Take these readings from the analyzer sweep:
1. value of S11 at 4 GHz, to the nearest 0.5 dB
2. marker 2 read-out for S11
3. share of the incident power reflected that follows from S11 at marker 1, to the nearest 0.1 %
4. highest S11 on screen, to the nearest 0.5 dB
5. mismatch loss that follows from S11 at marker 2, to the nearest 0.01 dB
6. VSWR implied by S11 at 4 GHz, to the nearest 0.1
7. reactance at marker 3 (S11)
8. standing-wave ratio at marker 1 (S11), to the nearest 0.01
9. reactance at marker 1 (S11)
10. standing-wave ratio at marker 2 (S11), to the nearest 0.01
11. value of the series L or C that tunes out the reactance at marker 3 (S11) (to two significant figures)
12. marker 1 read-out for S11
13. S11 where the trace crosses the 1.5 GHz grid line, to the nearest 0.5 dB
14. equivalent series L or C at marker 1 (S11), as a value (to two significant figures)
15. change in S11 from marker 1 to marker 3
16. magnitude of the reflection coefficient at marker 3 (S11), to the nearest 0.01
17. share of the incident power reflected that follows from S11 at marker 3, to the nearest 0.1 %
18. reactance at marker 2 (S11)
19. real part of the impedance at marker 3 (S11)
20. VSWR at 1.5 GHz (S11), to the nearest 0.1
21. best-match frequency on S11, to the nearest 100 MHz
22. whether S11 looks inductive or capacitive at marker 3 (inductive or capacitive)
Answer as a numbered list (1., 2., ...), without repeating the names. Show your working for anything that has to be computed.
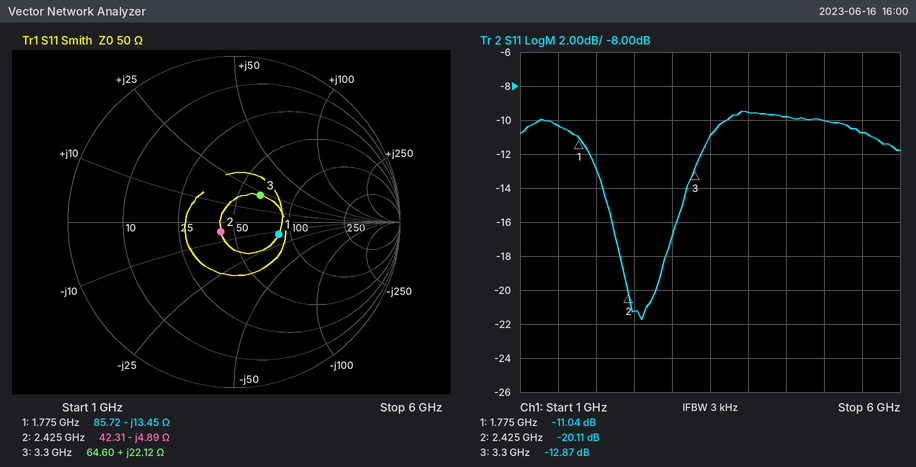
1. -9.5 dB
2. -20.11 dB
3. 10^(-11.04/10) ≈ 7.9 %
4. -9.5 dB
5. −10 log10(1 − 10^(-20.11/10)) ≈ 0.04 dB
6. |Γ| = 10^(-9.5/20) = 0.3350; VSWR = (1 + 0.3350)/(1 − 0.3350) ≈ 2.0
7. +22.12 Ω
8. 1.78
9. -13.45 Ω
10. 1.22
11. C = 1/(2π × 3.3 GHz × 22.12 Ω) ≈ 2.2 pF
12. -11.04 dB
13. -10.5 dB
14. C = 1/(2π × 1.775 GHz × 13.45 Ω) ≈ 6.7 pF
15. -12.87 − (-11.04) = -1.83 dB
16. 0.23
17. 10^(-12.87/10) ≈ 5.2 %
18. -4.89 Ω
19. 64.60 Ω
20. |Γ| = 10^(-10.5/20) = 0.2985; VSWR = (1 + 0.2985)/(1 − 0.2985) ≈ 1.9
21. 2.6 GHz
22. inductive
